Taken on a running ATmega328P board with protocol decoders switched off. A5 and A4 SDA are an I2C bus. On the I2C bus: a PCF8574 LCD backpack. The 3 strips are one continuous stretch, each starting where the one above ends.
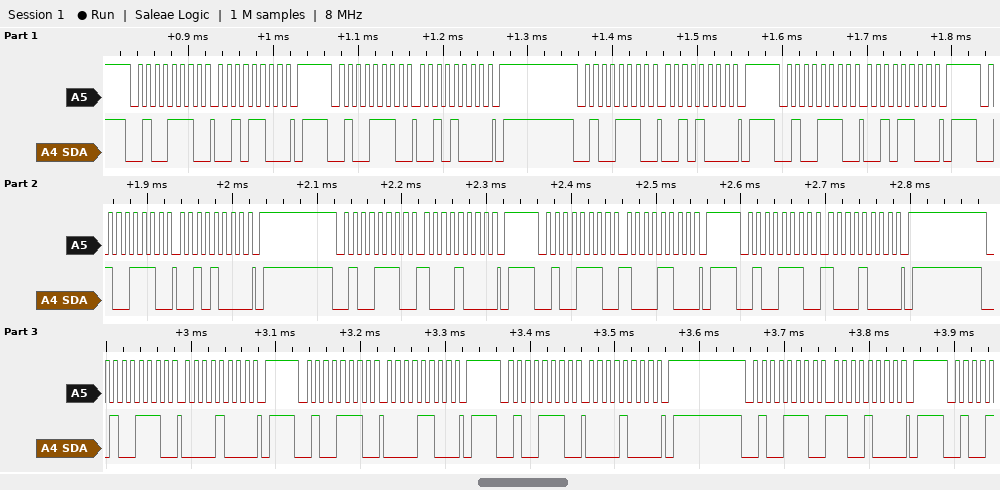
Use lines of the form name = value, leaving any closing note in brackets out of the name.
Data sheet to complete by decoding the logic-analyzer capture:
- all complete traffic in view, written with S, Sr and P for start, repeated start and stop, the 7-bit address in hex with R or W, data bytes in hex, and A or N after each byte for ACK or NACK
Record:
all complete traffic in view, written with S, Sr and P for start, repeated start and stop, the 7-bit address in hex with R or W, data bytes in hex, and A or N after each byte for ACK or NACK = S 27W A 2C A P S 27W A 28 A P S 27W A 28 A P S 27W A 2C A P S 27W A 28 A P S 27W A 88 A P S 27W A 8C A P S 27W A 88 A P S 27W A 08 A P S 27W A 0C A P S 27W A 08 A P S 27W A C8 A P
